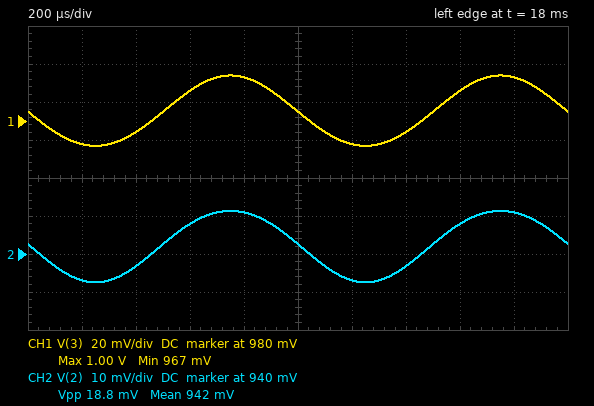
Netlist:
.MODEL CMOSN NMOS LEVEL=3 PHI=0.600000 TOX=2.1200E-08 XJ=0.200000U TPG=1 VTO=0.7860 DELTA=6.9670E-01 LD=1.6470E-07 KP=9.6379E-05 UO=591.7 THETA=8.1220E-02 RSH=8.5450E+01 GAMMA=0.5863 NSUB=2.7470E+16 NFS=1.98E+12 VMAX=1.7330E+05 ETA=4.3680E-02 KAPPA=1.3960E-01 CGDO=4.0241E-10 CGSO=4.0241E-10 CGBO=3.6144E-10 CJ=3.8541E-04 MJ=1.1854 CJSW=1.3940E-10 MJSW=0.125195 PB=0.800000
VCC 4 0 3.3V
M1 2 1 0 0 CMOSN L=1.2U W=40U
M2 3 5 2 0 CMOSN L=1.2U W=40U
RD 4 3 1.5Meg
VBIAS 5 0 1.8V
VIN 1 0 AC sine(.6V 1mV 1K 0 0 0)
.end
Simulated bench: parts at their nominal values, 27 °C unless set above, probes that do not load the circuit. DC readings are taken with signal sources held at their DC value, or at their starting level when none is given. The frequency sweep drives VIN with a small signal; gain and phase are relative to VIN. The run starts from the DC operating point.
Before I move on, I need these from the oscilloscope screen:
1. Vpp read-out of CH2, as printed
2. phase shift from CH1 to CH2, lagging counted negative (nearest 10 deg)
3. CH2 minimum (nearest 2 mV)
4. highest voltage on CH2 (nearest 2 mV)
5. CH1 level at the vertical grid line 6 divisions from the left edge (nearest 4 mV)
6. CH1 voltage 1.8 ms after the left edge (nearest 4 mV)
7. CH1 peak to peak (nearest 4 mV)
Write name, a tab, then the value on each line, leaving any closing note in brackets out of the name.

Vpp read-out of CH2, as printed	18.8 mV
phase shift from CH1 to CH2, lagging counted negative	0 deg
CH2 minimum	932 mV
highest voltage on CH2	952 mV
CH1 level at the vertical grid line 6 divisions from the left edge	968 mV
CH1 voltage 1.8 ms after the left edge	1.004 V
CH1 peak to peak	36 mV
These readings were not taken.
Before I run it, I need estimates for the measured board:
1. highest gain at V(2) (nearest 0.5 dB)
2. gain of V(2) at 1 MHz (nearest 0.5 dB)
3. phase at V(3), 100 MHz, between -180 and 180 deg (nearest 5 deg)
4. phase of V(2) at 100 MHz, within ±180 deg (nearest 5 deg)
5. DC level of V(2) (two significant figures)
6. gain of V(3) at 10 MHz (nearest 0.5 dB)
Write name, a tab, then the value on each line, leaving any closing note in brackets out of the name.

highest gain at V(2)	19.5 dB
gain of V(2) at 1 MHz	19.0 dB
phase at V(3), 100 MHz, between -180 and 180 deg	45 deg
phase of V(2) at 100 MHz, within ±180 deg	80 deg
DC level of V(2)	940 mV
gain of V(3) at 10 MHz	15.0 dB
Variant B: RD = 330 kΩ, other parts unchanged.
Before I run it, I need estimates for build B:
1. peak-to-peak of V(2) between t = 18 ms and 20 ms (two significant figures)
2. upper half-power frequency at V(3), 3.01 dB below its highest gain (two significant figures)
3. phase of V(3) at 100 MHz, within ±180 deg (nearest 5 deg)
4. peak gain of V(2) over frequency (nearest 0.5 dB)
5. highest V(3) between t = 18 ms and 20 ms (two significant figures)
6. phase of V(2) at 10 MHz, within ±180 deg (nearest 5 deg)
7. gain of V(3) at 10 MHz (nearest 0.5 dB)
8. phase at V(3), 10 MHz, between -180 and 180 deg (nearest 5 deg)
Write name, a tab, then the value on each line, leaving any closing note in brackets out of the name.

peak-to-peak of V(2) between t = 18 ms and 20 ms	1.9 mV
upper half-power frequency at V(3), 3.01 dB below its highest gain	25 MHz
phase of V(3) at 100 MHz, within ±180 deg	30 deg
peak gain of V(2) over frequency	-0.5 dB
highest V(3) between t = 18 ms and 20 ms	2.8 V
phase of V(2) at 10 MHz, within ±180 deg	165 deg
gain of V(3) at 10 MHz	15.0 dB
phase at V(3), 10 MHz, between -180 and 180 deg	150 deg
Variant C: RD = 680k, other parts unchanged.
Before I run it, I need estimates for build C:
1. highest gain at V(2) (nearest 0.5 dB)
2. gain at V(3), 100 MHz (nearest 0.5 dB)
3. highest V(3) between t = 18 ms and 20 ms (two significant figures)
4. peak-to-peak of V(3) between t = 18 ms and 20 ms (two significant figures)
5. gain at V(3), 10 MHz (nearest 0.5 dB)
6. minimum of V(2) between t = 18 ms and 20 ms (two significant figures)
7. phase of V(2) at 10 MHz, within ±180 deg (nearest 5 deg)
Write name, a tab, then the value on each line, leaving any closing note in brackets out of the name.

highest gain at V(2)	1.0 dB
gain at V(3), 100 MHz	1.5 dB
highest V(3) between t = 18 ms and 20 ms	2.2 V
peak-to-peak of V(3) between t = 18 ms and 20 ms	24 mV
gain at V(3), 10 MHz	19.5 dB
minimum of V(2) between t = 18 ms and 20 ms	990 mV
phase of V(2) at 10 MHz, within ±180 deg	160 deg
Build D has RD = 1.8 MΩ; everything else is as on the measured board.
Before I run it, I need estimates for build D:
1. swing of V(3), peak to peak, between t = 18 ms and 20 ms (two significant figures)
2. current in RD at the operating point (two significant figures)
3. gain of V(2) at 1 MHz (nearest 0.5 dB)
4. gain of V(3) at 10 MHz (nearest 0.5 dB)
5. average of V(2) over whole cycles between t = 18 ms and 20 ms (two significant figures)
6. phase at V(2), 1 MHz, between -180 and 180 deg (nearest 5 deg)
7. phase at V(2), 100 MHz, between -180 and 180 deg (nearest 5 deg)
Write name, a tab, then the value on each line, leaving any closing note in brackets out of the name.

swing of V(3), peak to peak, between t = 18 ms and 20 ms	30 mV
current in RD at the operating point	1.4 µA
gain of V(2) at 1 MHz	22.0 dB
gain of V(3) at 10 MHz	8.0 dB
average of V(2) over whole cycles between t = 18 ms and 20 ms	740 mV
phase at V(2), 1 MHz, between -180 and 180 deg	150 deg
phase at V(2), 100 MHz, between -180 and 180 deg	60 deg
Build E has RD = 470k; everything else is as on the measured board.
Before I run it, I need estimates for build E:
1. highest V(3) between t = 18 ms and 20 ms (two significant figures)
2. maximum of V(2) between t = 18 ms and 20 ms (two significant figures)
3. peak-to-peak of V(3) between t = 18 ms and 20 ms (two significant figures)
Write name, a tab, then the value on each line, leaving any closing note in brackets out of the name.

highest V(3) between t = 18 ms and 20 ms	2.6 V
maximum of V(2) between t = 18 ms and 20 ms	1.0 V
peak-to-peak of V(3) between t = 18 ms and 20 ms	17 mV
